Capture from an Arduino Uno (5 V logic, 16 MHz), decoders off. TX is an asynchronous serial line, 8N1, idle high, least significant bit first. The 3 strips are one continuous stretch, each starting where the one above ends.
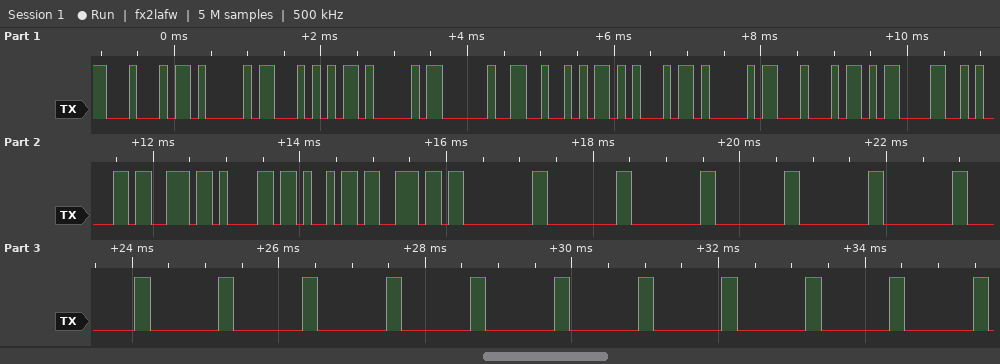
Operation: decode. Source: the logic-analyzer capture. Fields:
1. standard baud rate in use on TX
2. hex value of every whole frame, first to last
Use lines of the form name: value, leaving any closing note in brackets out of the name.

standard baud rate in use on TX: 9600 baud
hex value of every whole frame, first to last: 0x44 0x41 0x54 0x41 0x20 0x52 0x45 0x41 0x44 0x0D 0x0A 0x73 0x61 0x69 0x6E 0x00 0x00 0x00 0x00 0x00 0x00 0x00 0x00 0x00 0x00 0x00 0x00 0x00 0x00 0x00 0x00 0x00
